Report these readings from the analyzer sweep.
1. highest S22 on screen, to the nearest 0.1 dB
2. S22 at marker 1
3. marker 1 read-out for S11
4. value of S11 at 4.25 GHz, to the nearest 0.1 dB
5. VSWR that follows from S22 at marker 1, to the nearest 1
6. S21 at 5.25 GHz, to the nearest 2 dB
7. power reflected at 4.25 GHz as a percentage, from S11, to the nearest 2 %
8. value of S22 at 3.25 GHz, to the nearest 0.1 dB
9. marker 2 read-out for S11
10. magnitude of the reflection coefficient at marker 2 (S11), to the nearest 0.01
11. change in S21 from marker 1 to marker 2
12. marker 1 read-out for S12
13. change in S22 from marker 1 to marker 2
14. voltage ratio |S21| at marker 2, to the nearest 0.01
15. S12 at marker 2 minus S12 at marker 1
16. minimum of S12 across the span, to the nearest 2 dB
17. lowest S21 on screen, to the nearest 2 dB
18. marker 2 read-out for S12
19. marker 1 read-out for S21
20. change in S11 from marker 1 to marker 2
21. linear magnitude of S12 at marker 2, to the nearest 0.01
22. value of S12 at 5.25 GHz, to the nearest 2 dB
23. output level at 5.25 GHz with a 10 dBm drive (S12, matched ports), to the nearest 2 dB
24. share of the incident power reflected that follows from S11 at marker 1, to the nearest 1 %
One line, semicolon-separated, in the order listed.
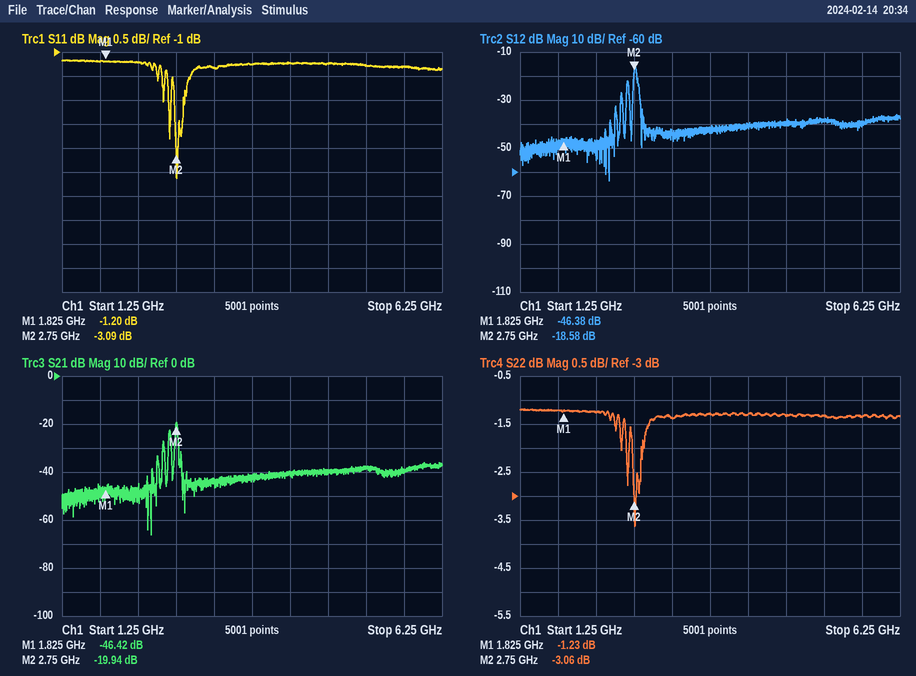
-1.2 dB; -1.23 dB; -1.20 dB; -1.2 dB; 14; -38 dB; 76 %; -1.4 dB; -3.09 dB; 0.70; 26.48 dB; -46.38 dB; -1.83 dB; 0.10; 27.80 dB; -64 dB; -66 dB; -18.58 dB; -46.42 dB; -1.89 dB; 0.12; -38 dB; -28 dBm; 76 %
